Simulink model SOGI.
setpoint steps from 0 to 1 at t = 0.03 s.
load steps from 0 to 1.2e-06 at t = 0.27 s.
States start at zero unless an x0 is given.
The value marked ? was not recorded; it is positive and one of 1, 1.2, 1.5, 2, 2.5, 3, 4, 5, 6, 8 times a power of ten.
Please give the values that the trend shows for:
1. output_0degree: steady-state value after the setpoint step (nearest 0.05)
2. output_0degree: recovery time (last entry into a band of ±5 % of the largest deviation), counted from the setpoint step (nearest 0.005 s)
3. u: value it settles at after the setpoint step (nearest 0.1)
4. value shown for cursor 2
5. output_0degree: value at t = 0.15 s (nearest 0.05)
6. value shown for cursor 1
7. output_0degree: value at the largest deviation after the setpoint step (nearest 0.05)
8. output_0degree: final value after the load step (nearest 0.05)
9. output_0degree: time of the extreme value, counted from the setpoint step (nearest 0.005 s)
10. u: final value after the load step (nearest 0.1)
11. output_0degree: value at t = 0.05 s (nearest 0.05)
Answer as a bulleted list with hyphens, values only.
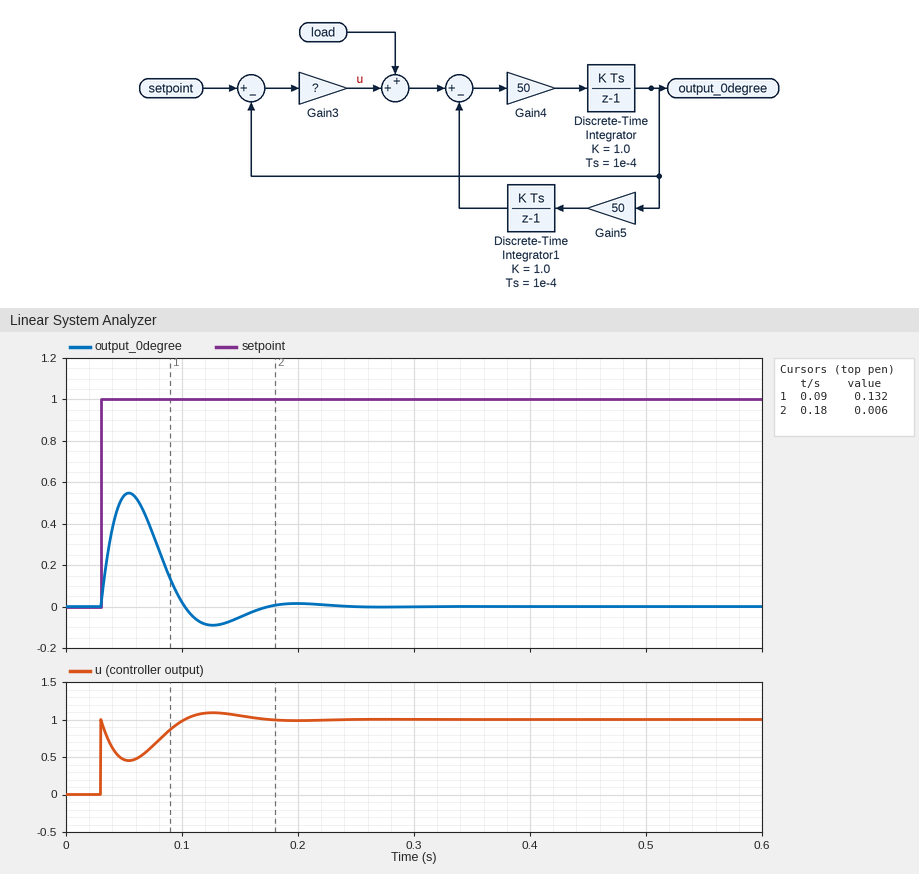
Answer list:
- 0.00
- 0.130 s
- 1.0
- 0.006
- -0.05
- 0.132
- 0.55
- 0.00
- 0.025 s
- 1.0
- 0.55
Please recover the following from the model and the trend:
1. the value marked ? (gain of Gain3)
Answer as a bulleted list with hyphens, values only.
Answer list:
- 1
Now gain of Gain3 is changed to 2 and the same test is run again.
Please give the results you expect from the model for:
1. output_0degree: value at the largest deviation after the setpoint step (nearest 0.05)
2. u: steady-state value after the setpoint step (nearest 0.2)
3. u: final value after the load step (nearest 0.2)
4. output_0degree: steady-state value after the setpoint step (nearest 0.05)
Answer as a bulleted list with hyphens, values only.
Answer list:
- 0.75
- 2.0
- 2.0
- 0.00
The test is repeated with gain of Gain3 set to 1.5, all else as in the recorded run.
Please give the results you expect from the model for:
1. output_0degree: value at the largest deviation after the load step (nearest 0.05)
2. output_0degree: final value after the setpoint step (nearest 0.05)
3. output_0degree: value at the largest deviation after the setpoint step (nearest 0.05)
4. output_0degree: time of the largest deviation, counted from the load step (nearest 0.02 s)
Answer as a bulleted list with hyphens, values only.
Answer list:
- 0.00
- 0.00
- 0.65
- 0.06 s
